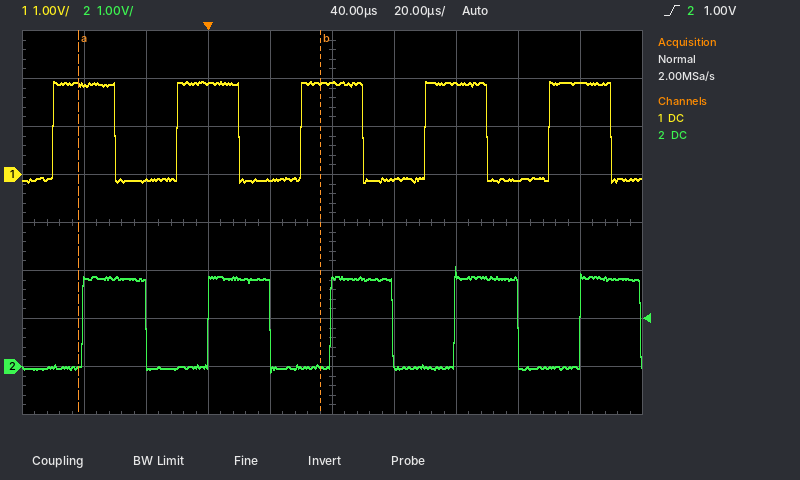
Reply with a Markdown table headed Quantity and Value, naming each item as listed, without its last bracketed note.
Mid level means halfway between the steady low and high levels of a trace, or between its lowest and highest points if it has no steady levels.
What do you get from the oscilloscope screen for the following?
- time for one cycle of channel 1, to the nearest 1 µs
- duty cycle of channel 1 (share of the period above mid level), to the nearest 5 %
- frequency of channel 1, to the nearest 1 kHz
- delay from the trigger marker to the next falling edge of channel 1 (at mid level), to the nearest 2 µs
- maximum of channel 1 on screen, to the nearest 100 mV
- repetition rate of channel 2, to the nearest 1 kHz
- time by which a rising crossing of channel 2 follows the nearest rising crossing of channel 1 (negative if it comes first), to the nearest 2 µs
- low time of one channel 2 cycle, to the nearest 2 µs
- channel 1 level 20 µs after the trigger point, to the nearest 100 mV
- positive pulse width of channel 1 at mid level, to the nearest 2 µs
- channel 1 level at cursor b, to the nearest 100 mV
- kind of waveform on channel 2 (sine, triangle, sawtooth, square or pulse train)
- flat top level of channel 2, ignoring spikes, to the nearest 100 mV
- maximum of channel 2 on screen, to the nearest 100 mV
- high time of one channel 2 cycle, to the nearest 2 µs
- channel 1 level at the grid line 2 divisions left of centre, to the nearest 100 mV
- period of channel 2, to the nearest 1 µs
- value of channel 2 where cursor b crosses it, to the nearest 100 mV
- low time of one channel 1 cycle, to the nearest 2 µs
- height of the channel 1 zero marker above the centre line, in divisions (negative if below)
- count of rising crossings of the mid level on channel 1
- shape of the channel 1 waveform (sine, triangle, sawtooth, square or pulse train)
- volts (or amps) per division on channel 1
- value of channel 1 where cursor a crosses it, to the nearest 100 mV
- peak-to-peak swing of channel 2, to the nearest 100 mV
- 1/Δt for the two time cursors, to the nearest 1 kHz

| Quantity | Value |
|---|---|
| time for one cycle of channel 1, to the nearest 1 µs | 40 µs |
| duty cycle of channel 1 (share of the period above mid level), to the nearest 5 % | 50 % |
| frequency of channel 1, to the nearest 1 kHz | 25 kHz |
| delay from the trigger marker to the next falling edge of channel 1 (at mid level), to the nearest 2 µs | 10 µs |
| maximum of channel 1 on screen, to the nearest 100 mV | 1.9 V |
| repetition rate of channel 2, to the nearest 1 kHz | 25 kHz |
| time by which a rising crossing of channel 2 follows the nearest rising crossing of channel 1 (negative if it comes first), to the nearest 2 µs | +10 µs |
| low time of one channel 2 cycle, to the nearest 2 µs | 20 µs |
| channel 1 level 20 µs after the trigger point, to the nearest 100 mV | -100 mV |
| positive pulse width of channel 1 at mid level, to the nearest 2 µs | 20 µs |
| channel 1 level at cursor b, to the nearest 100 mV | 1.9 V |
| kind of waveform on channel 2 | square |
| flat top level of channel 2, ignoring spikes, to the nearest 100 mV | 1.8 V |
| maximum of channel 2 on screen, to the nearest 100 mV | 2.1 V |
| high time of one channel 2 cycle, to the nearest 2 µs | 20 µs |
| channel 1 level at the grid line 2 divisions left of centre, to the nearest 100 mV | 1.9 V |
| period of channel 2, to the nearest 1 µs | 40 µs |
| value of channel 2 where cursor b crosses it, to the nearest 100 mV | 0.0 V |
| low time of one channel 1 cycle, to the nearest 2 µs | 20 µs |
| height of the channel 1 zero marker above the centre line, in divisions | +1.0 div |
| count of rising crossings of the mid level on channel 1 | 5 |
| shape of the channel 1 waveform | square |
| volts (or amps) per division on channel 1 | 1 V |
| value of channel 1 where cursor a crosses it, to the nearest 100 mV | 1.9 V |
| peak-to-peak swing of channel 2, to the nearest 100 mV | 2.2 V |
| 1/Δt for the two time cursors, to the nearest 1 kHz | 13 kHz |
